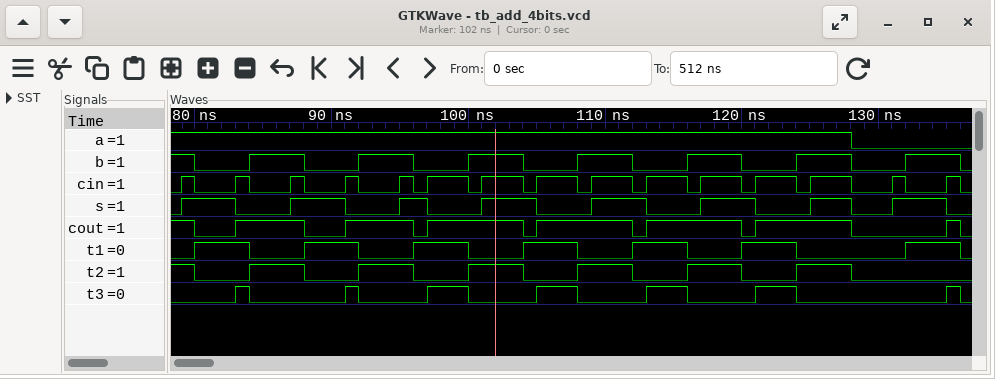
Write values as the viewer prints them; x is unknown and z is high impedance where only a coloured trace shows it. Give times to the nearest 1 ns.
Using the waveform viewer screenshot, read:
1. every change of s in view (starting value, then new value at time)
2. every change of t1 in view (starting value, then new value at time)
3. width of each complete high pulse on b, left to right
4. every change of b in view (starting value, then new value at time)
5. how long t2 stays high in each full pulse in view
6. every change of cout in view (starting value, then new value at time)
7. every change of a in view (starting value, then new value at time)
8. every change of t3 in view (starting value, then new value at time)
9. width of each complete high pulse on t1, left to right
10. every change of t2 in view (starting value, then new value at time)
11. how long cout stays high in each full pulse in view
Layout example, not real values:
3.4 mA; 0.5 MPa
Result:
0, 1 at 79 ns, 0 at 83 ns, 1 at 87 ns, 0 at 91 ns, 1 at 95 ns, 0 at 97 ns, 1 at 101 ns, 0 at 105 ns, 1 at 109 ns, 0 at 113 ns, 1 at 117 ns, 0 at 121 ns, 1 at 125 ns, 0 at 128 ns, 1 at 131 ns, 0 at 135 ns; 0, 1 at 80 ns, 0 at 84 ns, 1 at 88 ns, 0 at 92 ns, 1 at 96 ns, 0 at 100 ns, 1 at 104 ns, 0 at 108 ns, 1 at 112 ns, 0 at 116 ns, 1 at 120 ns, 0 at 124 ns, 1 at 132 ns, 0 at 136 ns; 4 ns, 4 ns, 4 ns, 4 ns, 4 ns, 4 ns, 4 ns; 1, 0 at 80 ns, 1 at 84 ns, 0 at 88 ns, 1 at 92 ns, 0 at 96 ns, 1 at 100 ns, 0 at 104 ns, 1 at 108 ns, 0 at 112 ns, 1 at 116 ns, 0 at 120 ns, 1 at 124 ns, 0 at 128 ns, 1 at 132 ns, 0 at 136 ns; 4 ns, 4 ns, 4 ns, 4 ns, 4 ns, 4 ns; 1, 0 at 80 ns, 1 at 83 ns, 0 at 88 ns, 1 at 91 ns, 0 at 96 ns, 1 at 97 ns, 0 at 104 ns, 1 at 105 ns, 0 at 112 ns, 1 at 113 ns, 0 at 120 ns, 1 at 121 ns, 0 at 128 ns, 1 at 135 ns, 0 at 136 ns; 1, 0 at 128 ns; 0, 1 at 83 ns, 0 at 84 ns, 1 at 91 ns, 0 at 92 ns, 1 at 97 ns, 0 at 100 ns, 1 at 105 ns, 0 at 108 ns, 1 at 113 ns, 0 at 116 ns, 1 at 121 ns, 0 at 124 ns, 1 at 135 ns, 0 at 136 ns; 4 ns, 4 ns, 4 ns, 4 ns, 4 ns, 4 ns, 4 ns; 1, 0 at 80 ns, 1 at 84 ns, 0 at 88 ns, 1 at 92 ns, 0 at 96 ns, 1 at 100 ns, 0 at 104 ns, 1 at 108 ns, 0 at 112 ns, 1 at 116 ns, 0 at 120 ns, 1 at 124 ns, 0 at 128 ns; 5 ns, 5 ns, 7 ns, 7 ns, 7 ns, 7 ns, 1 ns
